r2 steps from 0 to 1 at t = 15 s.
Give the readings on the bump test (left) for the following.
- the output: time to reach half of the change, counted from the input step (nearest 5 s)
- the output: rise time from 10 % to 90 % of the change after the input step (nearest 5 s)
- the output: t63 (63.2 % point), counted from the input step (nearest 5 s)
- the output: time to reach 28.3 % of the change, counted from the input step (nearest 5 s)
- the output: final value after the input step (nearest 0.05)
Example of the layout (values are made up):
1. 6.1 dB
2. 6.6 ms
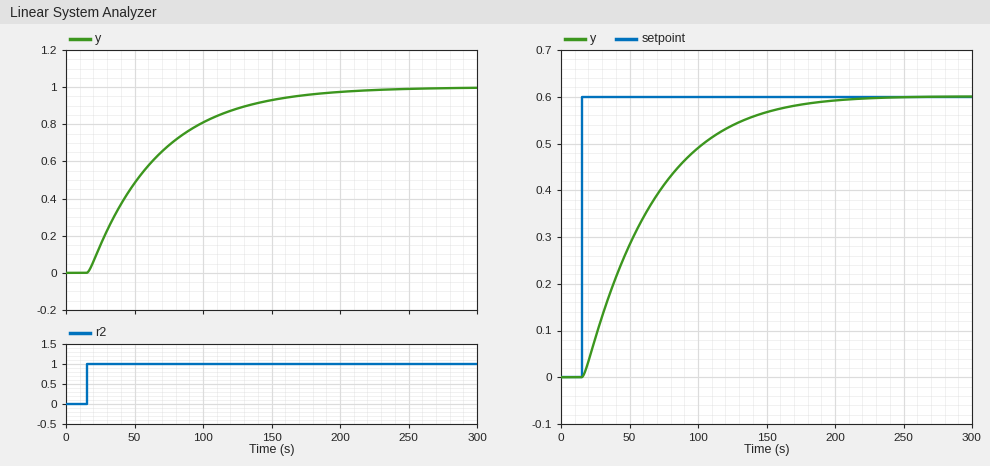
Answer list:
1. 35 s
2. 110 s
3. 50 s
4. 20 s
5. 1.00
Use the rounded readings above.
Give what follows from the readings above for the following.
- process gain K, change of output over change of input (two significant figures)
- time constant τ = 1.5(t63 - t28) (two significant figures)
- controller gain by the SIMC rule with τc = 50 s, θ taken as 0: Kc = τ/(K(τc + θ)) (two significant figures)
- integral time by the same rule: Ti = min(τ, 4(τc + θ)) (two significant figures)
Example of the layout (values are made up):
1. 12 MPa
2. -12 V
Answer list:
1. 1.0
2. 45 s
3. 0.90
4. 45 s
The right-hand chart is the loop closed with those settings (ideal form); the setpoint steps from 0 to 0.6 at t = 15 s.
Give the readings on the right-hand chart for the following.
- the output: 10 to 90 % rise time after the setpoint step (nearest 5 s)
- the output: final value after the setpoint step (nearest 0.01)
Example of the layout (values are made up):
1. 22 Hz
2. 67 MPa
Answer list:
1. 105 s
2. 0.60
